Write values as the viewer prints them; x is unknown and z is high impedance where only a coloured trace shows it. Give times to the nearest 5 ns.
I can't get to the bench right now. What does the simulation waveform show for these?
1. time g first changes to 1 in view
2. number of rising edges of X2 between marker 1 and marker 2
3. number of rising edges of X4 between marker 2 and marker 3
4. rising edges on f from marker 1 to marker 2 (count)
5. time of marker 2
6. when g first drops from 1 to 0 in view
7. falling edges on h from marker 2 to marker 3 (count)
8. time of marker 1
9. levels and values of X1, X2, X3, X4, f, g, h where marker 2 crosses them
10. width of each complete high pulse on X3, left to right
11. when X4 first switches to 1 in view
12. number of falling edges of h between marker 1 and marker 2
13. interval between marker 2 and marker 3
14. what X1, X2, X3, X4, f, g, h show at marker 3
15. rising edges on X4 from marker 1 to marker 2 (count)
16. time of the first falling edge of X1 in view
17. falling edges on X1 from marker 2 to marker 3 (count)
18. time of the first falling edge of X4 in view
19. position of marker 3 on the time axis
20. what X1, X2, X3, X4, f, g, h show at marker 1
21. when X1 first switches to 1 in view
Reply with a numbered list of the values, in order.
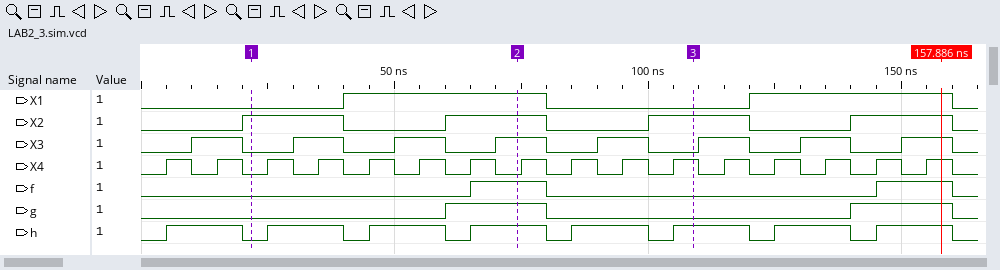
1. 60 ns
2. 1
3. 4
4. 1
5. 75 ns
6. 80 ns
7. 2
8. 20 ns
9. X1=1, X2=1, X3=1, X4=0, f=1, g=1, h=1
10. 10 ns, 10 ns, 10 ns, 10 ns, 10 ns, 10 ns, 10 ns, 10 ns
11. 5 ns
12. 2
13. 35 ns
14. X1=0, X2=1, X3=0, X4=1, f=0, g=0, h=1
15. 5
16. 80 ns
17. 1
18. 10 ns
19. 110 ns
20. X1=0, X2=1, X3=0, X4=0, f=0, g=0, h=0
21. 40 ns
